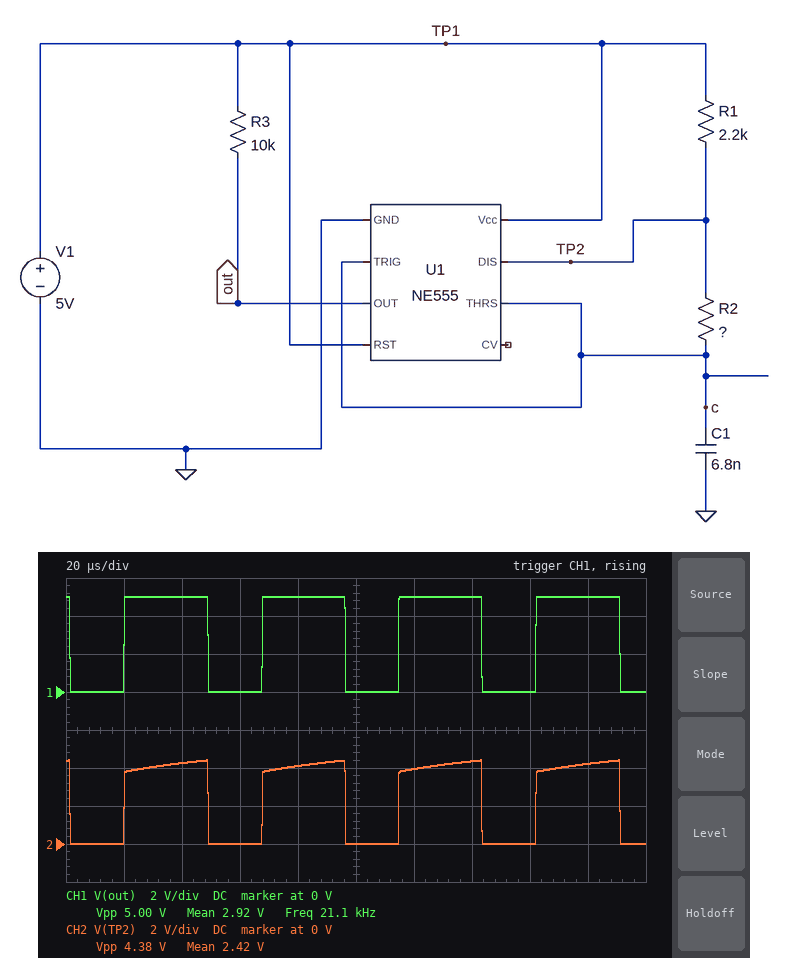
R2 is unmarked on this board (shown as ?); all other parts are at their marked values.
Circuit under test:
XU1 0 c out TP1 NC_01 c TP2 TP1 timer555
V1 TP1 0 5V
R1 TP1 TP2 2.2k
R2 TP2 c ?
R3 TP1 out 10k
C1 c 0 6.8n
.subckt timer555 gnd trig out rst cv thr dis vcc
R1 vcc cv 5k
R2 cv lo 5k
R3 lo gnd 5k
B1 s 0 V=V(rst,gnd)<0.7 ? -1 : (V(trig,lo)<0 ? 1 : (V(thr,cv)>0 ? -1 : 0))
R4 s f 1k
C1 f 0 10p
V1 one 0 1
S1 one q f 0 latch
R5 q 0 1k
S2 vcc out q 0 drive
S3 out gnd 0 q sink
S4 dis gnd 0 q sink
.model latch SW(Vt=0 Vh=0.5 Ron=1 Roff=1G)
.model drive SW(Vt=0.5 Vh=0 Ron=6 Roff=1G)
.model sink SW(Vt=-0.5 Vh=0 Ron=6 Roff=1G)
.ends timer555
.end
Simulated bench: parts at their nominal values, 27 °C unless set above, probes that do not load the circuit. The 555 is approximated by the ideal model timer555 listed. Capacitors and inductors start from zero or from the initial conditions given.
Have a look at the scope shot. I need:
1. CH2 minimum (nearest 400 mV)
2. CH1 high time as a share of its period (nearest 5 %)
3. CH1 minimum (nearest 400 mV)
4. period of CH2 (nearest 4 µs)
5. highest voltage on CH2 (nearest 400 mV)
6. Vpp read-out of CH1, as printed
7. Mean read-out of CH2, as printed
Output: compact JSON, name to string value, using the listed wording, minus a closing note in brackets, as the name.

{"CH2 minimum": "0 V", "CH1 high time as a share of its period": "60 %", "CH1 minimum": "0 V", "period of CH2": "48 µs", "highest voltage on CH2": "4.4 V", "Vpp read-out of CH1, as printed": "5.00 V", "Mean read-out of CH2, as printed": "2.42 V"}
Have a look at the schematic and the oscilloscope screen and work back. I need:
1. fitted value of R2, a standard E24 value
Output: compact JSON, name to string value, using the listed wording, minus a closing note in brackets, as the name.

{"fitted value of R2, a standard E24 value": "3.9 kΩ"}
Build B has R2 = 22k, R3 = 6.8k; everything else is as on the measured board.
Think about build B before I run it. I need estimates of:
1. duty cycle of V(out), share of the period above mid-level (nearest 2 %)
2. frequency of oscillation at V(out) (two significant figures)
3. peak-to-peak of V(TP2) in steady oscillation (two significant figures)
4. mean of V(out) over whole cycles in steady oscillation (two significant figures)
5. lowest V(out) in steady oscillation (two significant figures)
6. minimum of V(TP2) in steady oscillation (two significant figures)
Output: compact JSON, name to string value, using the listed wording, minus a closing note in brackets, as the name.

{"duty cycle of V(out), share of the period above mid-level": "52 %", "frequency of oscillation at V(out)": "4.6 kHz", "peak-to-peak of V(TP2) in steady oscillation": "4.8 V", "mean of V(out) over whole cycles in steady oscillation": "2.6 V", "lowest V(out) in steady oscillation": "4.4 mV", "minimum of V(TP2) in steady oscillation": "14 mV"}
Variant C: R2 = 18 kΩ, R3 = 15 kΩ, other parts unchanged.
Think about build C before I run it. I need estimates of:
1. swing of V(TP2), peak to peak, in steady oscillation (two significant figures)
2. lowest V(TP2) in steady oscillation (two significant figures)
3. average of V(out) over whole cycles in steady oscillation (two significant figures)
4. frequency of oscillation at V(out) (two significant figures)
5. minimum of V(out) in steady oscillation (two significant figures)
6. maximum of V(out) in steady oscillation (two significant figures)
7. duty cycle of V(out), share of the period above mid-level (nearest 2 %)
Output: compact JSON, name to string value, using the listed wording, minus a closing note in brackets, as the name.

{"swing of V(TP2), peak to peak, in steady oscillation": "4.8 V", "lowest V(TP2) in steady oscillation": "14 mV", "average of V(out) over whole cycles in steady oscillation": "2.6 V", "frequency of oscillation at V(out)": "5.5 kHz", "minimum of V(out) in steady oscillation": "2.0 mV", "maximum of V(out) in steady oscillation": "5.0 V", "duty cycle of V(out), share of the period above mid-level": "52 %"}
